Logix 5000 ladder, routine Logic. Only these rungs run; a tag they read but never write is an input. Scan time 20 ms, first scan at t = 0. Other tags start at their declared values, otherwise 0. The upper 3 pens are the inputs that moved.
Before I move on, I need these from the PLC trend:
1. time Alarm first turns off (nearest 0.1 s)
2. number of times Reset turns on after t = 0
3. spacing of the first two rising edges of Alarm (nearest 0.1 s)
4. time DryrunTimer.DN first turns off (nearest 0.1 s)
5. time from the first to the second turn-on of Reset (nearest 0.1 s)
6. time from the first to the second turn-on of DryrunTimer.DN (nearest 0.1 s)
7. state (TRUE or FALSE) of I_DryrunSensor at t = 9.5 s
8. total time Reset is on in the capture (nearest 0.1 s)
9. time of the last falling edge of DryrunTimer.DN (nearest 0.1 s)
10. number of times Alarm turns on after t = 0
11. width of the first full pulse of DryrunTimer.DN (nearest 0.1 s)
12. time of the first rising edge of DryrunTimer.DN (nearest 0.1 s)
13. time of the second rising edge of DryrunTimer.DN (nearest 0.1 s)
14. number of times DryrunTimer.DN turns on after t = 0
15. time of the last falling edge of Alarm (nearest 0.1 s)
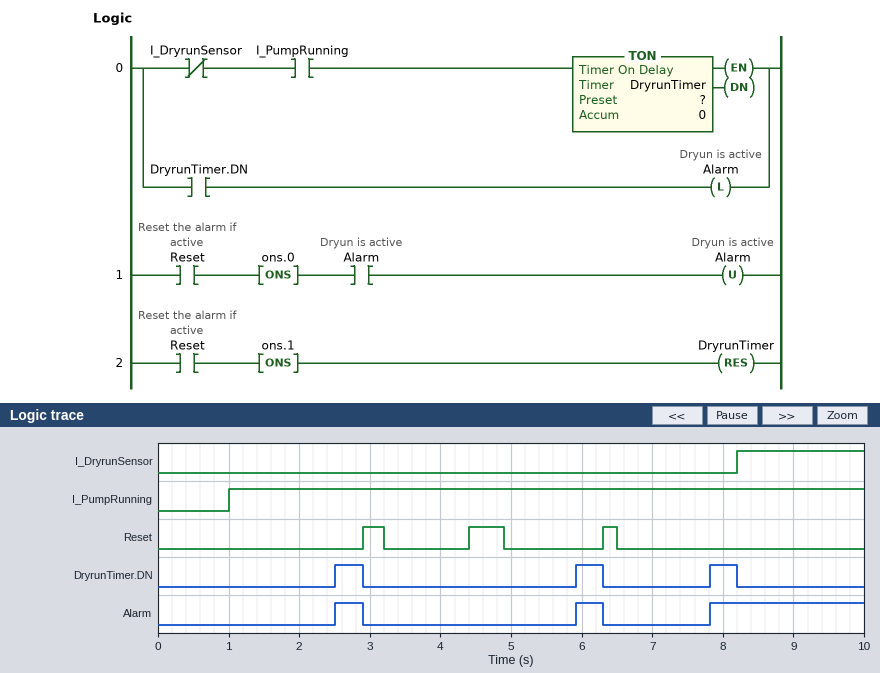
2.9 s
3
3.4 s
2.9 s
1.5 s
3.4 s
TRUE
1.0 s
8.2 s
3
0.4 s
2.5 s
5.9 s
3
6.3 s
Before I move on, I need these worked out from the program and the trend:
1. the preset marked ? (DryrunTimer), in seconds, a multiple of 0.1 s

1.5 s
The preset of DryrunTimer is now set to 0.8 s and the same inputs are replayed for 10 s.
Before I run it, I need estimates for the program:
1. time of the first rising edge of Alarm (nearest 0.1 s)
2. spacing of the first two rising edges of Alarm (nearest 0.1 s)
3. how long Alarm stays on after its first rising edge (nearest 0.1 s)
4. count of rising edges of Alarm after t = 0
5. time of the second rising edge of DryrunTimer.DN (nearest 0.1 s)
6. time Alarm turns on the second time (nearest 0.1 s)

1.8 s
1.9 s
1.1 s
4
3.7 s
3.7 s
